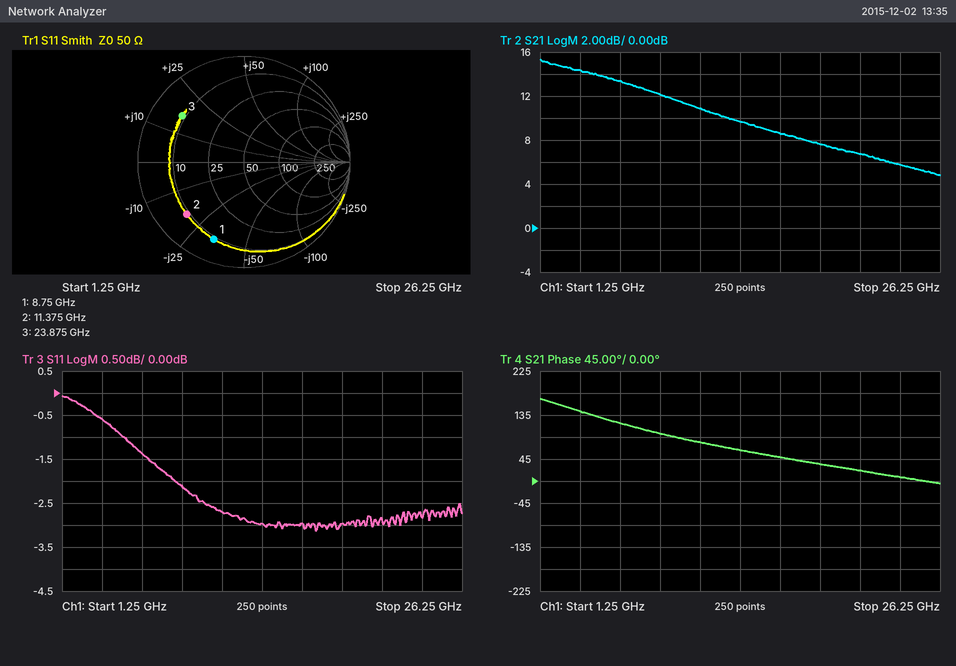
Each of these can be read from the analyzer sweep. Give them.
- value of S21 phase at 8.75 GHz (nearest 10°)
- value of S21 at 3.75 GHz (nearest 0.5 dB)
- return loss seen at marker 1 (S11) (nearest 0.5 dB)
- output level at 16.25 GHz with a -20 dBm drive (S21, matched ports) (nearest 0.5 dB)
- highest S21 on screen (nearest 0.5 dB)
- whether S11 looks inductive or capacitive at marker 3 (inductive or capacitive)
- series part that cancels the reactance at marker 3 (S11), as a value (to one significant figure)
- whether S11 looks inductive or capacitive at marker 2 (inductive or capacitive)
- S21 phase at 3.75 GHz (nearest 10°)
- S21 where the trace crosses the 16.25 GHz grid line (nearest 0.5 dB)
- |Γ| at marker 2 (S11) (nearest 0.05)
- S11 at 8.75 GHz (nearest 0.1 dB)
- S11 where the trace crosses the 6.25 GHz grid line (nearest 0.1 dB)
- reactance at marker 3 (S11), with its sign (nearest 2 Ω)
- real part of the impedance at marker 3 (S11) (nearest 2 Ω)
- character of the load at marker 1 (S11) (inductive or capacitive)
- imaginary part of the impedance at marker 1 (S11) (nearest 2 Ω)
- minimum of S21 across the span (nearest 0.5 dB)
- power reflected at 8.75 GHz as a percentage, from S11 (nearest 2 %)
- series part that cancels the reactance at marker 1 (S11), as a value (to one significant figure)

100°
14.5 dB
2.0 dB
-11.5 dBm
15.5 dB
inductive
400 fF
capacitive
140°
8.5 dB
0.75
-2.1 dB
-1.4 dB
+16 Ω
8 Ω
capacitive
-34 Ω
5.0 dB
62 %
600 pH
